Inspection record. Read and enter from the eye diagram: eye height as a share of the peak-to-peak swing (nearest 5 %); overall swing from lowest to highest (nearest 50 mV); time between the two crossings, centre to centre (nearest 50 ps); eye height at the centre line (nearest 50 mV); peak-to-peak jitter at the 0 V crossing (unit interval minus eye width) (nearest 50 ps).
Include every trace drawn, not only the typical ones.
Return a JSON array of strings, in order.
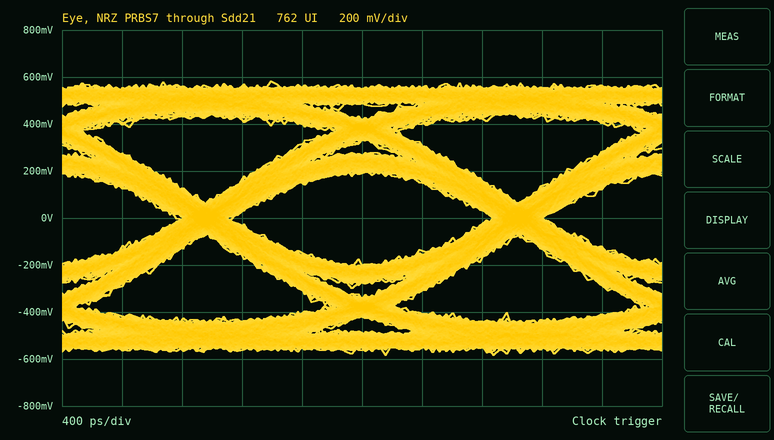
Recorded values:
["35 %", "1.15 V", "2.10 ns", "400 mV", "350 ps"]
